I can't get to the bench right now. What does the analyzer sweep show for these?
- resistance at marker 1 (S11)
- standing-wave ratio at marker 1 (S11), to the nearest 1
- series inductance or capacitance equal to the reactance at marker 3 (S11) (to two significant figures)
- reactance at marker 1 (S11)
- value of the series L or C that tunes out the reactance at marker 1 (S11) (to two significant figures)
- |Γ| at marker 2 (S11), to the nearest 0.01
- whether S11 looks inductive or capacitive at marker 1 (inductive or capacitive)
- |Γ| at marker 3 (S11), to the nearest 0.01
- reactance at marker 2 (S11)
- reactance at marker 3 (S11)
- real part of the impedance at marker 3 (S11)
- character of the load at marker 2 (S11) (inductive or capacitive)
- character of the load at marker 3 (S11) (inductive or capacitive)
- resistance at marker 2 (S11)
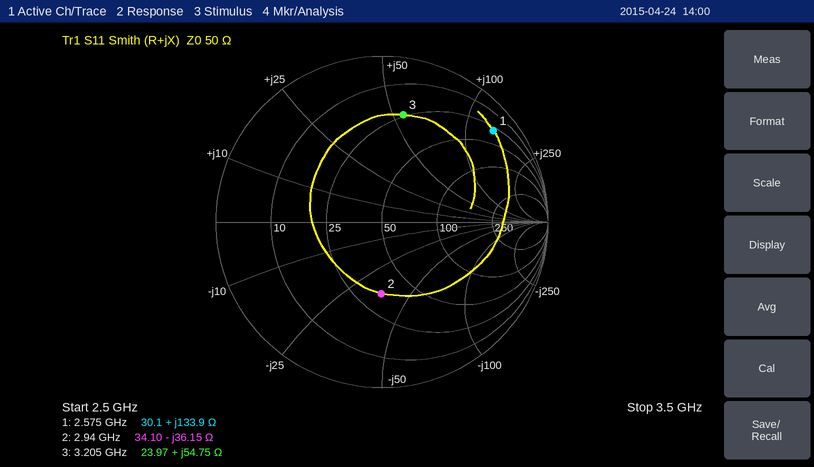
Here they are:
30.1 Ω
14
2.7 nH
+133.9 Ω
460 fF
0.43
inductive
0.66
-36.15 Ω
+54.75 Ω
23.97 Ω
capacitive
inductive
34.10 Ω
